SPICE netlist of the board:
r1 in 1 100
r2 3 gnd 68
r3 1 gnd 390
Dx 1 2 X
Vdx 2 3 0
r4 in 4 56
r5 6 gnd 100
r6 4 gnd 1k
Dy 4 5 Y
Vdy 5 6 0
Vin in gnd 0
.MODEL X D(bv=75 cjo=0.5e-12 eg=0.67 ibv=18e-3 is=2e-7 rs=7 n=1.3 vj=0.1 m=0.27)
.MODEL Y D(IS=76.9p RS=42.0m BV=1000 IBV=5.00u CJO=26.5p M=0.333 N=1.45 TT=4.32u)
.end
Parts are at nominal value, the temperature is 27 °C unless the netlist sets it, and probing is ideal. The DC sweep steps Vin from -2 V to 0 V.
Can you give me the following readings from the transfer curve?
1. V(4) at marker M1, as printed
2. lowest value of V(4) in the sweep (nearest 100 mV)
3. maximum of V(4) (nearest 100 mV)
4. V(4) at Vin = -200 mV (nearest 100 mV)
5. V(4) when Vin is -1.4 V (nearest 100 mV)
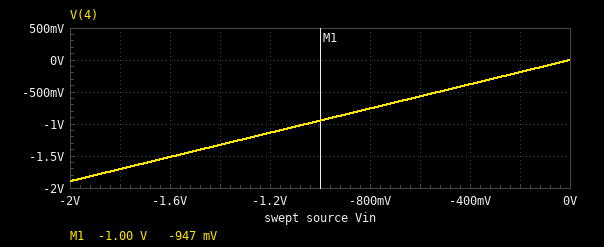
-947 mV
-1.9 V
0 V
-200 mV
-1.3 V
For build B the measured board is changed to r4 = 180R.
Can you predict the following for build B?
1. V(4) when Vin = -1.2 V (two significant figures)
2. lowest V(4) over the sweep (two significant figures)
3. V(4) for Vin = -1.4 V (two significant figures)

-1.0 V
-1.7 V
-1.2 V
